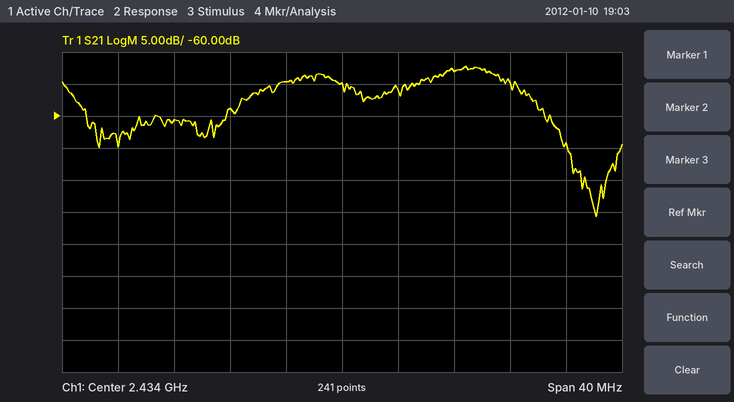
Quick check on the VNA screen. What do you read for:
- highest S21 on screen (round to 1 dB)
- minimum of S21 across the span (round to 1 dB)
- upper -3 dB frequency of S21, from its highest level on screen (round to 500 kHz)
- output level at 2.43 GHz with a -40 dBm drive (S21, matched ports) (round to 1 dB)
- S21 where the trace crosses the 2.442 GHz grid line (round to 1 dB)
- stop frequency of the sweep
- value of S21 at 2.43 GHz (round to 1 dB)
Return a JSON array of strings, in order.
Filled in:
["-52 dB", "-76 dB", "2.4460 GHz", "-95 dBm", "-53 dB", "2.454 GHz", "-55 dB"]
